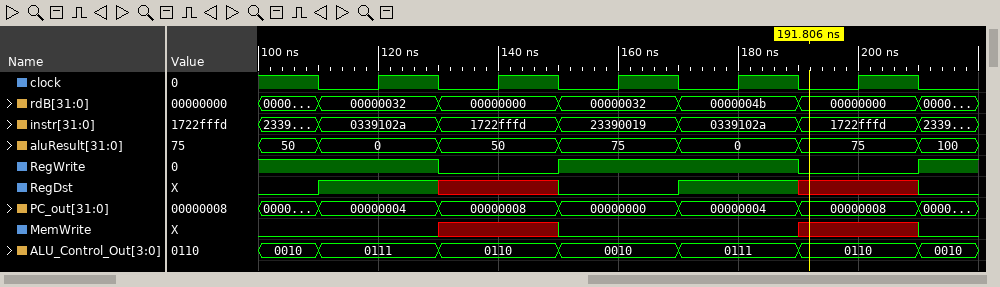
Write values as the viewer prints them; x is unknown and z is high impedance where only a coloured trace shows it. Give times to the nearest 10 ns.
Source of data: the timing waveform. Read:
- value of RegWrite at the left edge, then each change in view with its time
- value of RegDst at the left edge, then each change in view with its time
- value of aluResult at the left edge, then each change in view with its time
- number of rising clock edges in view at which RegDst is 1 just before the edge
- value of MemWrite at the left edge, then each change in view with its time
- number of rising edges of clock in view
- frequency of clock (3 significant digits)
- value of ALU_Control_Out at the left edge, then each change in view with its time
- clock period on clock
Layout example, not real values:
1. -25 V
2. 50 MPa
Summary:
1. 1, 0 at 130 ns, 1 at 150 ns, 0 at 190 ns, 1 at 210 ns
2. 0, 1 at 110 ns, x at 130 ns, 0 at 150 ns, 1 at 170 ns, x at 190 ns, 0 at 210 ns
3. 50, 0 at 110 ns, 50 at 130 ns, 75 at 150 ns, 0 at 170 ns, 75 at 190 ns, 100 at 210 ns
4. 2
5. 0, x at 130 ns, 0 at 150 ns, x at 190 ns, 0 at 210 ns
6. 5
7. 50.0 MHz
8. 0010, 0111 at 110 ns, 0110 at 130 ns, 0010 at 150 ns, 0111 at 170 ns, 0110 at 190 ns, 0010 at 210 ns
9. 20 ns
